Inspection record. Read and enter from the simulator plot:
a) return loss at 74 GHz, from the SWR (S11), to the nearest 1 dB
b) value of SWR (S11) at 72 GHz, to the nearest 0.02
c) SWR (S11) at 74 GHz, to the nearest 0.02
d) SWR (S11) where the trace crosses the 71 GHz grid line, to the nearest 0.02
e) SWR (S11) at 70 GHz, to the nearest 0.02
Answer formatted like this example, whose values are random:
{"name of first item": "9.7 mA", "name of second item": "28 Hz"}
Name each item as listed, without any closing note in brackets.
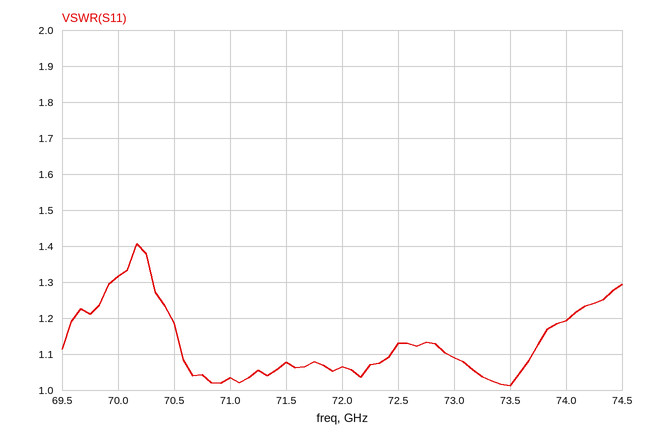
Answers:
{"return loss at 74 GHz, from the SWR (S11), to the nearest 1 dB": "21 dB", "value of SWR (S11) at 72 GHz, to the nearest 0.02": "1.06", "SWR (S11) at 74 GHz, to the nearest 0.02": "1.20", "SWR (S11) where the trace crosses the 71 GHz grid line, to the nearest 0.02": "1.04", "SWR (S11) at 70 GHz, to the nearest 0.02": "1.32"}
